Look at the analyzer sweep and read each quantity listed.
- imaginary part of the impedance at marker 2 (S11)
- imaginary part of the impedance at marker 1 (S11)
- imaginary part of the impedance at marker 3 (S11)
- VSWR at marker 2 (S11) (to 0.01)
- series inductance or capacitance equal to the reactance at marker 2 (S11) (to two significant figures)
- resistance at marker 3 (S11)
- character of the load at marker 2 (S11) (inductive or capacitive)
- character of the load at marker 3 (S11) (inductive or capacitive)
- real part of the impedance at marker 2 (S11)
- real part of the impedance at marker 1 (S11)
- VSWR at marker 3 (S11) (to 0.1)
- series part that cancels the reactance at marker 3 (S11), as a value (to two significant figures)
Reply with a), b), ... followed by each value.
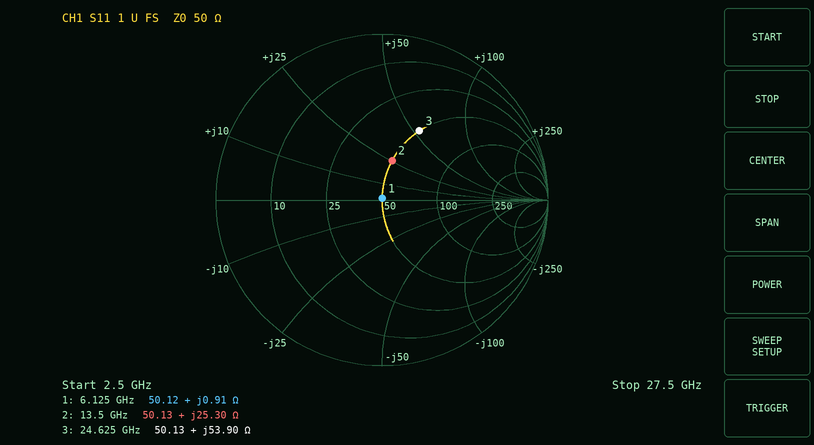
a) +25.30 Ω
b) +0.91 Ω
c) +53.90 Ω
d) 1.65
e) 300 pH
f) 50.13 Ω
g) inductive
h) inductive
i) 50.13 Ω
j) 50.12 Ω
k) 2.8
l) 120 fF
